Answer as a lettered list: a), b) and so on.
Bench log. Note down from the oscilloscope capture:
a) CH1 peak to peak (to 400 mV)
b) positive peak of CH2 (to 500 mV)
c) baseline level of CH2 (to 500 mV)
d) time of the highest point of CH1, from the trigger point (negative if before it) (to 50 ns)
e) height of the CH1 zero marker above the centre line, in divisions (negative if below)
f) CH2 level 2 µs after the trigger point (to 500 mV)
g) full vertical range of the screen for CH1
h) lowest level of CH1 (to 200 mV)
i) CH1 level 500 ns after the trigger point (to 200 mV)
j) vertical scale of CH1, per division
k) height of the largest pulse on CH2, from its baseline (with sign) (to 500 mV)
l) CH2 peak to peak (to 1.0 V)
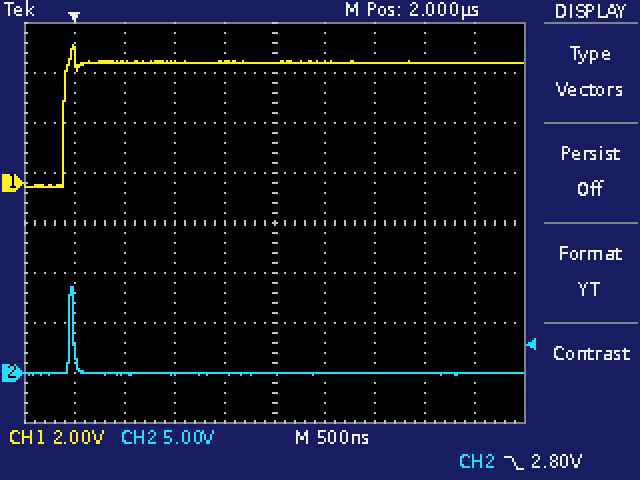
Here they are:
a) 5.6 V
b) 8.5 V
c) 0.0 V
d) 0 ns
e) +0.8 div
f) 0.0 V
g) 16 V
h) -200 mV
i) 4.8 V
j) 2 V
k) +8.5 V
l) 9.0 V
